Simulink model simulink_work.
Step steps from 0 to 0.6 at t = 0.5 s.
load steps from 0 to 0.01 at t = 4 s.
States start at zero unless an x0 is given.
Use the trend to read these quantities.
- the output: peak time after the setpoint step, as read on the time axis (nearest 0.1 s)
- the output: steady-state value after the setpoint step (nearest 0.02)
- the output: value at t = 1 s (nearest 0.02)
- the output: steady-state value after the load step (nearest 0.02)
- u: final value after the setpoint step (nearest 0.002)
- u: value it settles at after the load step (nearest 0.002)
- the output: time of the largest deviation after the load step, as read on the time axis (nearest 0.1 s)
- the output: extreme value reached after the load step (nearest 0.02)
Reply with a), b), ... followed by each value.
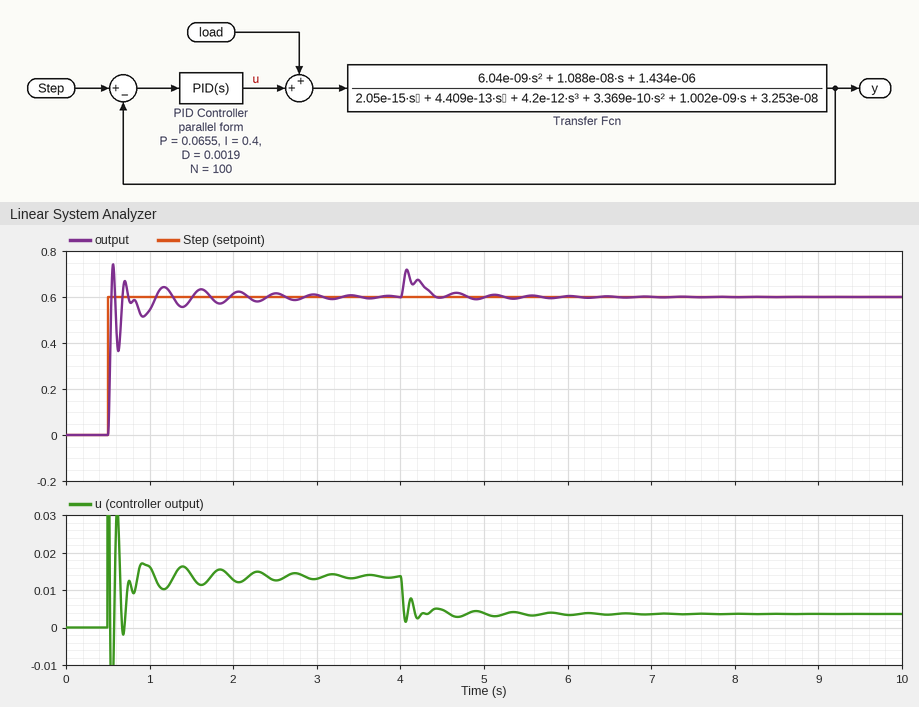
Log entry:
a) 0.6 s
b) 0.60
c) 0.54
d) 0.60
e) 0.014
f) 0.004
g) 4.1 s
h) 0.72
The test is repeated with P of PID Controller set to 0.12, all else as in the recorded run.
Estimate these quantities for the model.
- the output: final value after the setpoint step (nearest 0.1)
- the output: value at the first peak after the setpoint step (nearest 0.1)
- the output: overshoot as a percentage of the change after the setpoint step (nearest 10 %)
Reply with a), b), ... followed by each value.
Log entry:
a) 0.6
b) 0.9
c) 50 %
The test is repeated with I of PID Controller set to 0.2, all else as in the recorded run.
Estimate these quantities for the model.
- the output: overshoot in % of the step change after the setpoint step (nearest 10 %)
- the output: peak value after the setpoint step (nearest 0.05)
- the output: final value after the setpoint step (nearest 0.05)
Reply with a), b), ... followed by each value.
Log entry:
a) 20 %
b) 0.70
c) 0.60
